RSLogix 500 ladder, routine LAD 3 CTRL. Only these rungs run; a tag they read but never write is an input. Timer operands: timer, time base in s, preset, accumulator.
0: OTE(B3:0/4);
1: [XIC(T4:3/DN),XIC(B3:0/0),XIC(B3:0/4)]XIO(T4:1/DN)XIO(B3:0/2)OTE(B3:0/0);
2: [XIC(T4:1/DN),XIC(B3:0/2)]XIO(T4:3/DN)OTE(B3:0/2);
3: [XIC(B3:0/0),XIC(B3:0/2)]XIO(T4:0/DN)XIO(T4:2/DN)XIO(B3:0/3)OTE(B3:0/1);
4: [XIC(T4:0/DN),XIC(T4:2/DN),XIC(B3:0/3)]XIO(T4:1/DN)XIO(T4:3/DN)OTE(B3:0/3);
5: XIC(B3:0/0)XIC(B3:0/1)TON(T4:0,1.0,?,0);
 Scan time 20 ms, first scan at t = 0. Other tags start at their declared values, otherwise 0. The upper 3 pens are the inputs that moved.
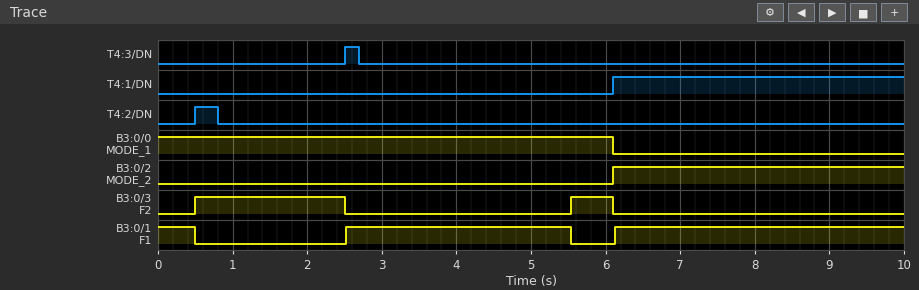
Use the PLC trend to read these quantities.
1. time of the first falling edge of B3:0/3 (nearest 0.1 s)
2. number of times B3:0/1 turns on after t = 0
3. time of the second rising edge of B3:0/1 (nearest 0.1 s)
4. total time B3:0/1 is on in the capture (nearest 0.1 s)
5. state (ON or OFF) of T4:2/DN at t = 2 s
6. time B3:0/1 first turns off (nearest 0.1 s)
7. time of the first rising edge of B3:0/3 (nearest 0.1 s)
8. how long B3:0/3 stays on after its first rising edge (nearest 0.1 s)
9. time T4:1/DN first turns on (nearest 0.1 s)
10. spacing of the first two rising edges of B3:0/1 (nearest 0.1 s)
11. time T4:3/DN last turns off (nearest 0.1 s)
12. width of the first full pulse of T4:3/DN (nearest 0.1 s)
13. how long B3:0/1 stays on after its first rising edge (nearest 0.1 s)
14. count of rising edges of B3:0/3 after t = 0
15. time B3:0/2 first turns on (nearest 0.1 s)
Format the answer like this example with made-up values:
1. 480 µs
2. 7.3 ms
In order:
1. 2.5 s
2. 2
3. 6.1 s
4. 7.4 s
5. OFF
6. 0.5 s
7. 0.5 s
8. 2.0 s
9. 6.1 s
10. 3.6 s
11. 2.7 s
12. 0.2 s
13. 3.0 s
14. 2
15. 6.1 s
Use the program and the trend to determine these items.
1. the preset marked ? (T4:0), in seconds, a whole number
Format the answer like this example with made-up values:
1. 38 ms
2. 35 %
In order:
1. 3 s
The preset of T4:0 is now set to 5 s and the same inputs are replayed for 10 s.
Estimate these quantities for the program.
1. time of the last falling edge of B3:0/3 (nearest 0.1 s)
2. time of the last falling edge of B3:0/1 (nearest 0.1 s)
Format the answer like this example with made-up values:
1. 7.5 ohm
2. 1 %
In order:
1. 2.5 s
2. 0.5 s
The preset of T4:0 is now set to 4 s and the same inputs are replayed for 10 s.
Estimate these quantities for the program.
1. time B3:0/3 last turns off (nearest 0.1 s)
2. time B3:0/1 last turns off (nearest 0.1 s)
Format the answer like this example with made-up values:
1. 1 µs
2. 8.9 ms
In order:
1. 2.5 s
2. 0.5 s
